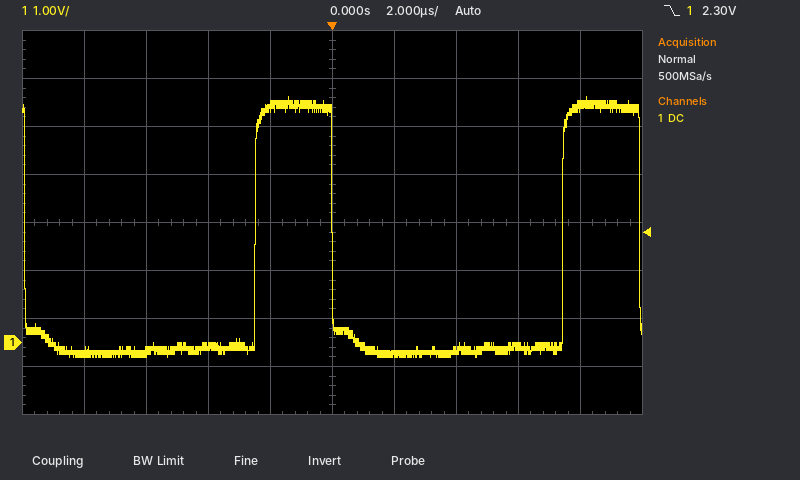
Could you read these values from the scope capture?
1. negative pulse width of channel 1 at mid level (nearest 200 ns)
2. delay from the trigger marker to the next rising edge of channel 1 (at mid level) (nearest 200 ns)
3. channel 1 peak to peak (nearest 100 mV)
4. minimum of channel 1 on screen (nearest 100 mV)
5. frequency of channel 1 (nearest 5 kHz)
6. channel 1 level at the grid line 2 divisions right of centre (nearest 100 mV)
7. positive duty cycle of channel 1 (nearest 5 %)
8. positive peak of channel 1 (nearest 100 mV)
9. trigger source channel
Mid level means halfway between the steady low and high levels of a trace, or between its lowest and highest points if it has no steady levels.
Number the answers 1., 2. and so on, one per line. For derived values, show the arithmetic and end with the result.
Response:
1. 7.4 µs
2. 7.4 µs
3. 5.1 V − (-300 mV) = 5.4 V
4. -300 mV
5. 100 kHz
6. -200 mV
7. 25 %
8. 5.1 V
9. channel 1
